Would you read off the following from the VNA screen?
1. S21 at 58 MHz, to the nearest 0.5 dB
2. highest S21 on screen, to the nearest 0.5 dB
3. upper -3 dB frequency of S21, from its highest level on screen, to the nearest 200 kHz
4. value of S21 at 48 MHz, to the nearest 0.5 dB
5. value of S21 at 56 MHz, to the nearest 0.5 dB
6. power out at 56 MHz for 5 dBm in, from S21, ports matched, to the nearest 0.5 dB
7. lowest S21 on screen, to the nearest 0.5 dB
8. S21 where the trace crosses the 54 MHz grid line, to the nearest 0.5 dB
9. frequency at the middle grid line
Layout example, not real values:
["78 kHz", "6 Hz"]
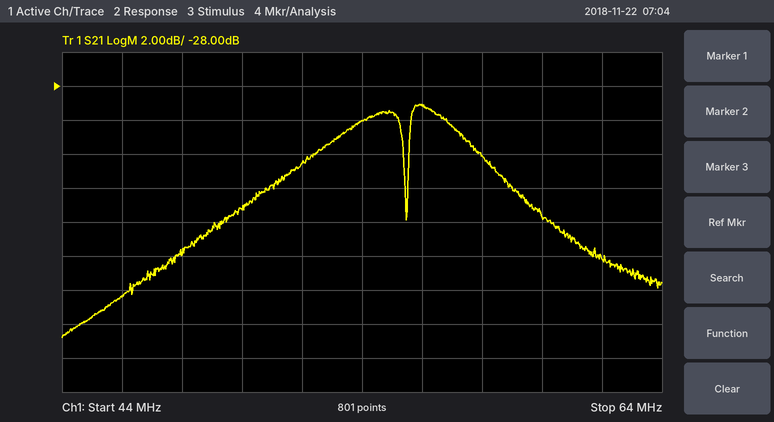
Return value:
["-32.0 dB", "-29.0 dB", "58.0 MHz", "-38.0 dB", "-29.0 dB", "-24.0 dBm", "-43.0 dB", "-30.0 dB", "54 MHz"]
